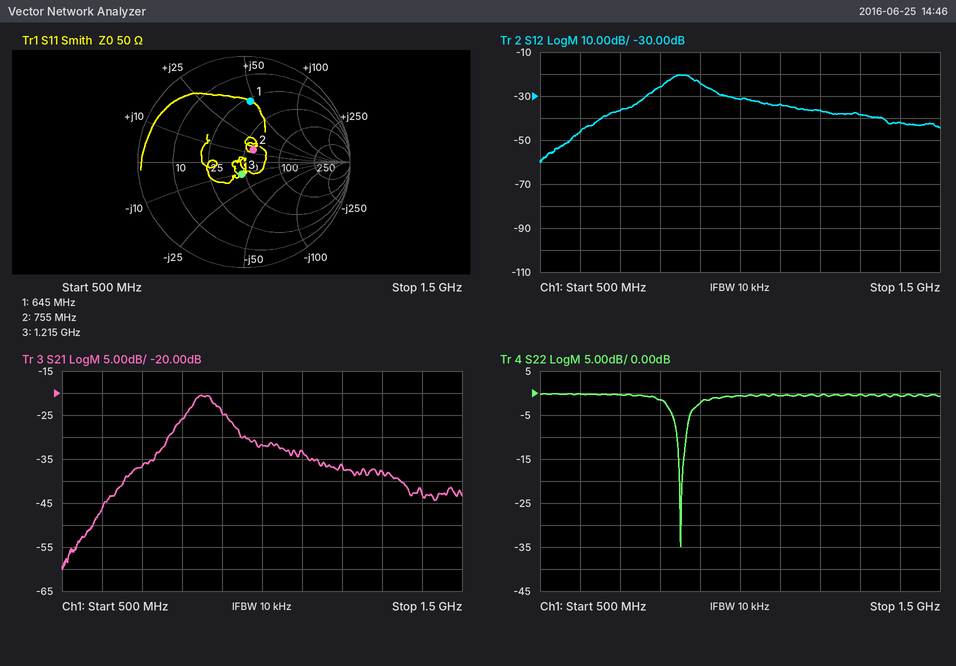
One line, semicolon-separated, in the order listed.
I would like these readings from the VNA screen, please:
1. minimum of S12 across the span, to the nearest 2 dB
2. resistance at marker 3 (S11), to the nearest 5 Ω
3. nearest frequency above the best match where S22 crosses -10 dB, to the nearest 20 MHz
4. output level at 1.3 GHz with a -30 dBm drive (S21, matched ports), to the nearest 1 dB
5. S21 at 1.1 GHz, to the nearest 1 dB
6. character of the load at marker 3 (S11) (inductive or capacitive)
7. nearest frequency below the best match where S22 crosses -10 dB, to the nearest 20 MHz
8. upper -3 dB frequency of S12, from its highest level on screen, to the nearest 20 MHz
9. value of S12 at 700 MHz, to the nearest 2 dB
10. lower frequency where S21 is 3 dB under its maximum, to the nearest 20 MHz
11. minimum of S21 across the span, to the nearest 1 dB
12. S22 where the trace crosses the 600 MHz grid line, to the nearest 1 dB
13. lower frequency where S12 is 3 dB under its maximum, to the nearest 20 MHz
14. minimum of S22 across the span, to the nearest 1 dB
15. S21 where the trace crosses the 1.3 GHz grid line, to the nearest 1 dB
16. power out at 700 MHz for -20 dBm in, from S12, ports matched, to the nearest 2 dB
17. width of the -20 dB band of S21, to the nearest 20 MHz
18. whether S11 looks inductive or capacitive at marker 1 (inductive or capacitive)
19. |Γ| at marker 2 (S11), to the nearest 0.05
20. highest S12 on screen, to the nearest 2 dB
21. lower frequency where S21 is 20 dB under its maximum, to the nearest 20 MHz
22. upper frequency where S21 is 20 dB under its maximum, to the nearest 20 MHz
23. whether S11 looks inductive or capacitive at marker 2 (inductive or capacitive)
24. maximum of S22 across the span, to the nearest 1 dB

-60 dB; 45 Ω; 860 MHz; -68 dBm; -33 dB; capacitive; 840 MHz; 900 MHz; -36 dB; 820 MHz; -60 dB; 0 dB; 820 MHz; -35 dB; -38 dB; -56 dBm; 700 MHz; inductive; 0.15; -20 dB; 660 MHz; 1.36 GHz; inductive; 0 dB
